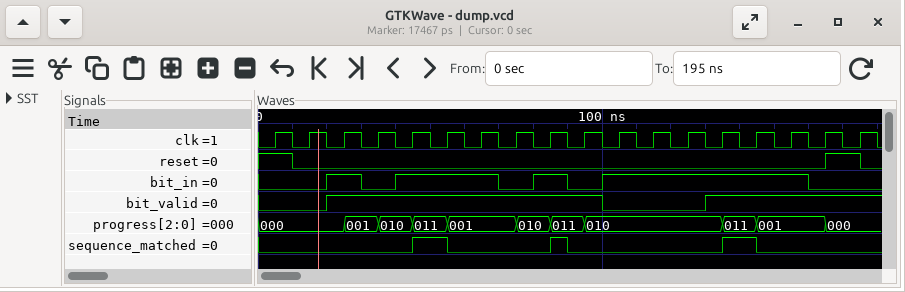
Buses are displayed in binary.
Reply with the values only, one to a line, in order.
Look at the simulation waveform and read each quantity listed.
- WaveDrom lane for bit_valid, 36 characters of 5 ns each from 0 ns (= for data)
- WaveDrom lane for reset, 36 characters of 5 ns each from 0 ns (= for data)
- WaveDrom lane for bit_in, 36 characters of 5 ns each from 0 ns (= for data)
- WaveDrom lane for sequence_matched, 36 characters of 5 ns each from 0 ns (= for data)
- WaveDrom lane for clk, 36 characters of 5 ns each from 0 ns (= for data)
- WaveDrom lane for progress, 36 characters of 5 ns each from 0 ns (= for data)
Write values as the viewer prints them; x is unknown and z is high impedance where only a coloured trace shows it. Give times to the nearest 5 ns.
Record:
{name: 'bit_valid', wave: '0...1...............0.....1.........'}
{name: 'reset', wave: '1.0..............................1.0'}
{name: 'bit_in', wave: '0...1.0.1.....0.1.0.1...........0...'}
{name: 'sequence_matched', wave: '0........1.0.....10........1.0......'}
{name: 'clk', wave: '010101010101010101010101010101010101'}
{name: 'progress', wave: '=....=.=.=.=...=.=.=.......=.=...=..', data: '000 001 010 011 001 010 011 010 011 001 000'}
